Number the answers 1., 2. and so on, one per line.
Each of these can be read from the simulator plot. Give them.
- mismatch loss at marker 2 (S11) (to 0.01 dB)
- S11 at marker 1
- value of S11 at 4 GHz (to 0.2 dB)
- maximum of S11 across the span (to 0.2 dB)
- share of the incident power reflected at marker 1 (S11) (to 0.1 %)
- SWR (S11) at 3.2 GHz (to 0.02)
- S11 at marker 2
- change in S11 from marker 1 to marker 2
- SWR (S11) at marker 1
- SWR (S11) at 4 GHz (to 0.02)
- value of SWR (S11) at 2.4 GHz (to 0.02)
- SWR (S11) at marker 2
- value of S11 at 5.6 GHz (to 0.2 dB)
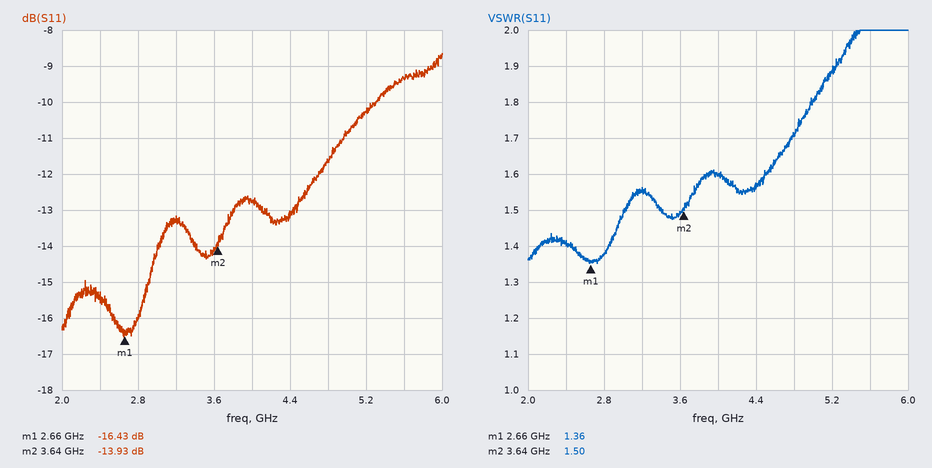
1. 0.18 dB
2. -16.43 dB
3. -12.8 dB
4. -8.6 dB
5. 2.3 %
6. 1.56
7. -13.93 dB
8. 2.50 dB
9. 1.36
10. 1.60
11. 1.40
12. 1.50
13. -9.4 dB
